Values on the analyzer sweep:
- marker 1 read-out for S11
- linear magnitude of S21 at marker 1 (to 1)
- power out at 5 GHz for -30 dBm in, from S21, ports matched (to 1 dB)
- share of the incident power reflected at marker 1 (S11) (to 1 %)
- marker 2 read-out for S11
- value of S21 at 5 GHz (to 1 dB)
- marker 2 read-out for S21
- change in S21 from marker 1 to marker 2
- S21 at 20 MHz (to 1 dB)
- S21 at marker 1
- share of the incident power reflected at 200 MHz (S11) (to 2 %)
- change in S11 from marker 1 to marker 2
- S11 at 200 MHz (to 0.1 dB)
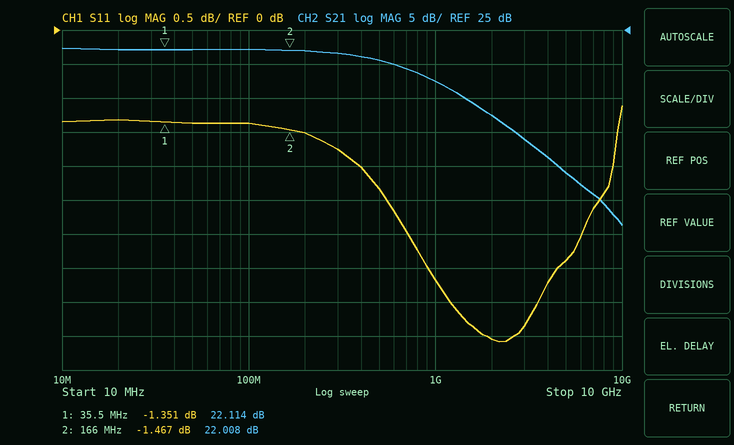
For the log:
-1.351 dB
13
-26 dBm
73 %
-1.467 dB
4 dB
22.008 dB
-0.106 dB
22 dB
22.114 dB
70 %
-0.116 dB
-1.5 dB
